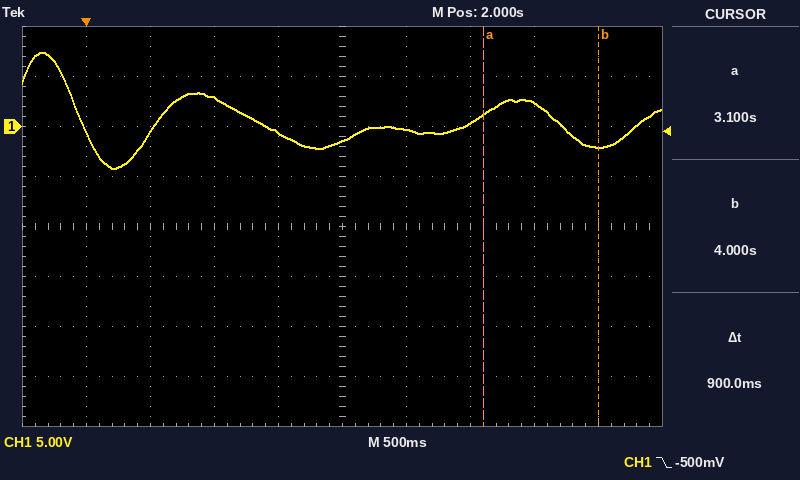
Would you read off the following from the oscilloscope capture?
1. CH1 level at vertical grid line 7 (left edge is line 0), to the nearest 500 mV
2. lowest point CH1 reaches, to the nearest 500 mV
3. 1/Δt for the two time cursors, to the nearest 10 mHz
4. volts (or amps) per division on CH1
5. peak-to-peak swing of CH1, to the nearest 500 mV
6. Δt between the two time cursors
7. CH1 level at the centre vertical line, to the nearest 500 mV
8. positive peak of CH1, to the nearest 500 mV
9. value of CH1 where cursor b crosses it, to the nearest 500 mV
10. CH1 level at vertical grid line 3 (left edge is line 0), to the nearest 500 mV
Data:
500 mV
-4.0 V
1.11 Hz
5 V
11.5 V
900 ms
-1.5 V
7.5 V
-2.0 V
3.0 V
